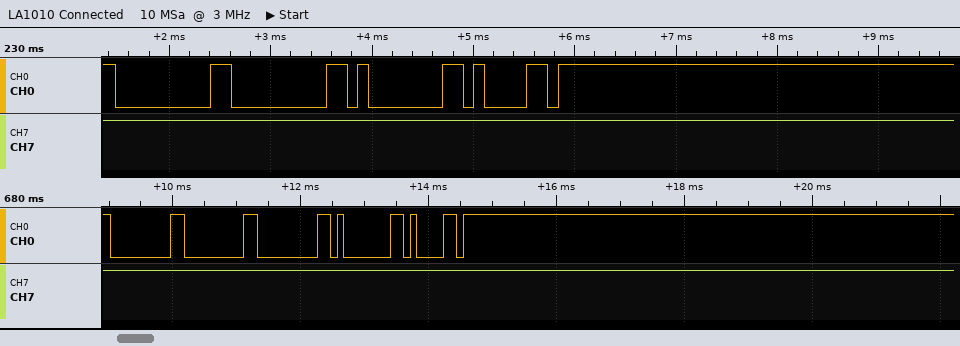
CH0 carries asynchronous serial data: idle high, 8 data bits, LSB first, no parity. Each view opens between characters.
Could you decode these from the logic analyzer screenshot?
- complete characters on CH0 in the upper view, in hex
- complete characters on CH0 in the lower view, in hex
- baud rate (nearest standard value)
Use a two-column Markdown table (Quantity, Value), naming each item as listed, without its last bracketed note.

| Quantity | Value |
|---|---|
| complete characters on CH0 in the upper view, in hex | 00, 00, 01, 61 |
| complete characters on CH0 in the lower view, in hex | 00, 00, 00, 01, 61 |
| baud rate | 9600 baud |
